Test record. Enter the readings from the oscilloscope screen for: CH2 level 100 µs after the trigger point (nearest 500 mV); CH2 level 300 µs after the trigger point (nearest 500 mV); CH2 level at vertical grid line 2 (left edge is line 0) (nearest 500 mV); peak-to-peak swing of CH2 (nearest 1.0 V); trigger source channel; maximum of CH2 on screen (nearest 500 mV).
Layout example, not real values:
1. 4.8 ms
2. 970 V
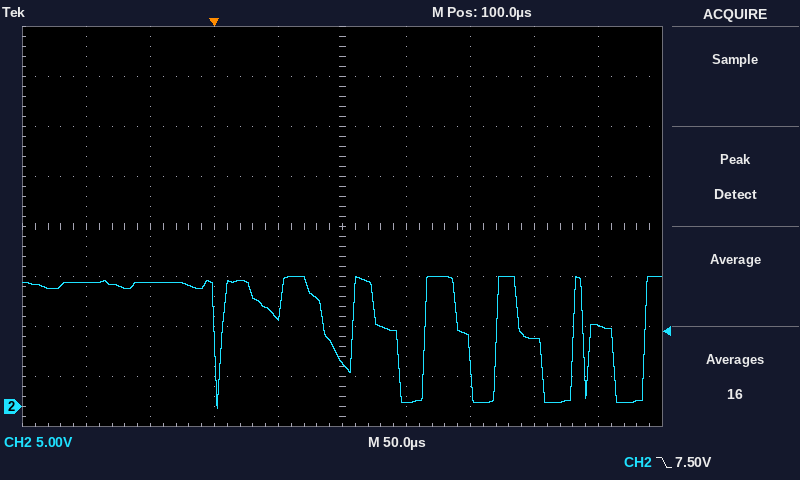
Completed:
1. 4.5 V
2. 8.0 V
3. 12.5 V
4. 13.0 V
5. CH2
6. 13.0 V
